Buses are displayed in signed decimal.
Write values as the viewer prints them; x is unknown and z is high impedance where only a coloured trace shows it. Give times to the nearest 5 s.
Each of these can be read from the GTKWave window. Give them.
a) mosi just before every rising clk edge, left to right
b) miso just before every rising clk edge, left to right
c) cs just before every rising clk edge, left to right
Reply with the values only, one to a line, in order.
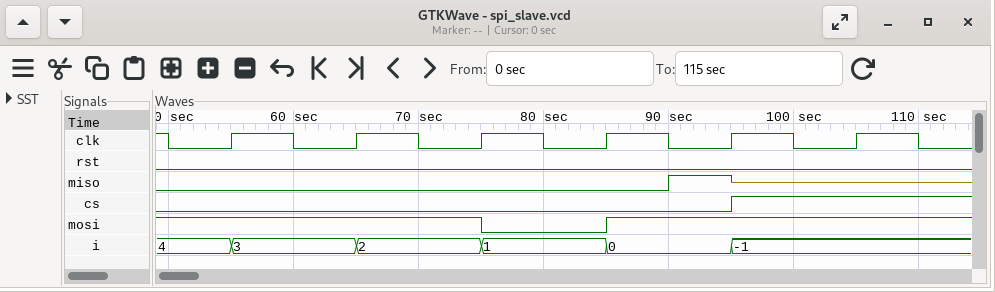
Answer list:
1 1 1 0 1 1
0 0 0 0 1 z
0 0 0 0 0 1
